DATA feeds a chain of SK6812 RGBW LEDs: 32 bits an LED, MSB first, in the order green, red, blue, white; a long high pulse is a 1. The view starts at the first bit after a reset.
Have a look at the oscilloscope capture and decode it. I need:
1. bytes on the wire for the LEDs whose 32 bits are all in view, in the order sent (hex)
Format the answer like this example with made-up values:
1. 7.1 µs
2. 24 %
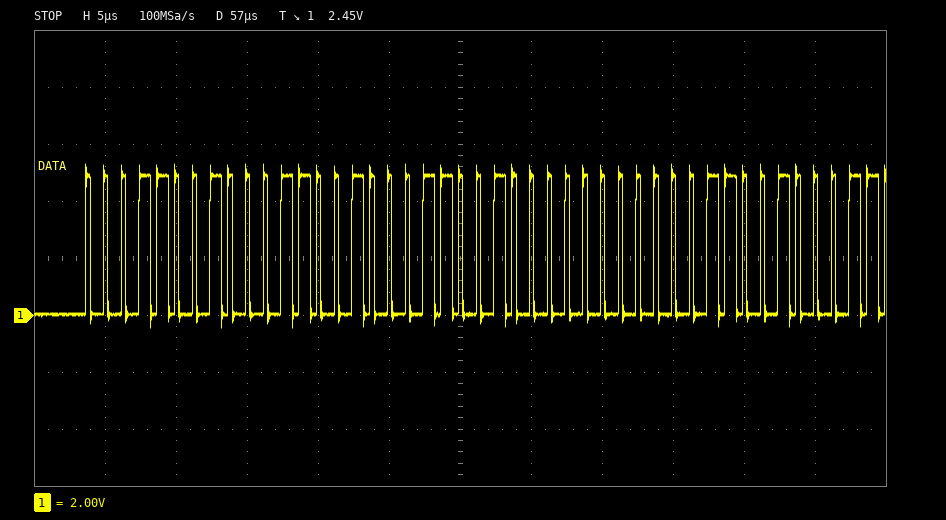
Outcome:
1. 19 19 19 00
